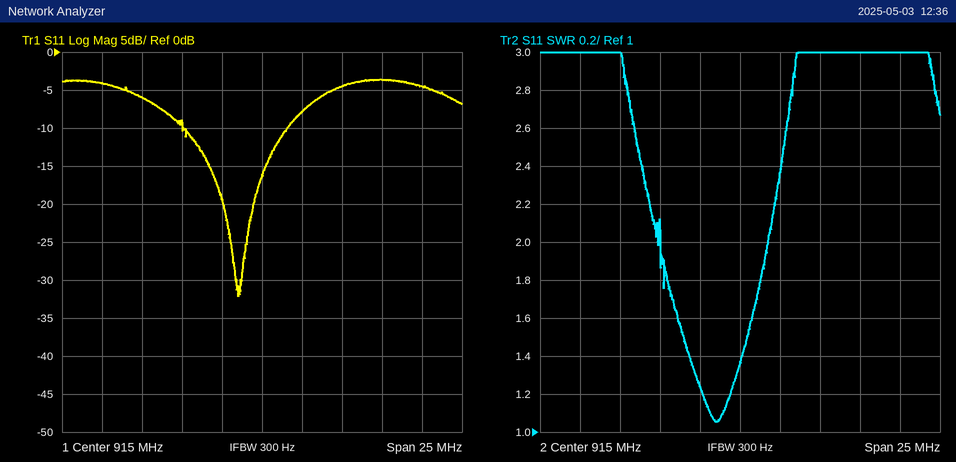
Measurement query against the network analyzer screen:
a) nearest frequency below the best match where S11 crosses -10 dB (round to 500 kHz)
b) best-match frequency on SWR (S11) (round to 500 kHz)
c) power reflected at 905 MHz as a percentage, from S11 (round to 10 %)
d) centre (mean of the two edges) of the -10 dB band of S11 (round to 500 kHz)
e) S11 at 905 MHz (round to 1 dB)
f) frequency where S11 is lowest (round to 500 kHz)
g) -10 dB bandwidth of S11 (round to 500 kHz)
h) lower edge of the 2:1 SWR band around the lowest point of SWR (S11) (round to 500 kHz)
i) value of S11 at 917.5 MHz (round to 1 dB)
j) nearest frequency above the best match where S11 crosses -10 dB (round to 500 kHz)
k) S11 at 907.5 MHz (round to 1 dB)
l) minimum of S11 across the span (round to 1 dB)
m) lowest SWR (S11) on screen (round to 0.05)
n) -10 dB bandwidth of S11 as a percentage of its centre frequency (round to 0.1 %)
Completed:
910.0 MHz
913.5 MHz
40 %
913.5 MHz
-4 dB
913.5 MHz
6.5 MHz
910.0 MHz
-8 dB
916.5 MHz
-6 dB
-32 dB
1.05
0.7 %
